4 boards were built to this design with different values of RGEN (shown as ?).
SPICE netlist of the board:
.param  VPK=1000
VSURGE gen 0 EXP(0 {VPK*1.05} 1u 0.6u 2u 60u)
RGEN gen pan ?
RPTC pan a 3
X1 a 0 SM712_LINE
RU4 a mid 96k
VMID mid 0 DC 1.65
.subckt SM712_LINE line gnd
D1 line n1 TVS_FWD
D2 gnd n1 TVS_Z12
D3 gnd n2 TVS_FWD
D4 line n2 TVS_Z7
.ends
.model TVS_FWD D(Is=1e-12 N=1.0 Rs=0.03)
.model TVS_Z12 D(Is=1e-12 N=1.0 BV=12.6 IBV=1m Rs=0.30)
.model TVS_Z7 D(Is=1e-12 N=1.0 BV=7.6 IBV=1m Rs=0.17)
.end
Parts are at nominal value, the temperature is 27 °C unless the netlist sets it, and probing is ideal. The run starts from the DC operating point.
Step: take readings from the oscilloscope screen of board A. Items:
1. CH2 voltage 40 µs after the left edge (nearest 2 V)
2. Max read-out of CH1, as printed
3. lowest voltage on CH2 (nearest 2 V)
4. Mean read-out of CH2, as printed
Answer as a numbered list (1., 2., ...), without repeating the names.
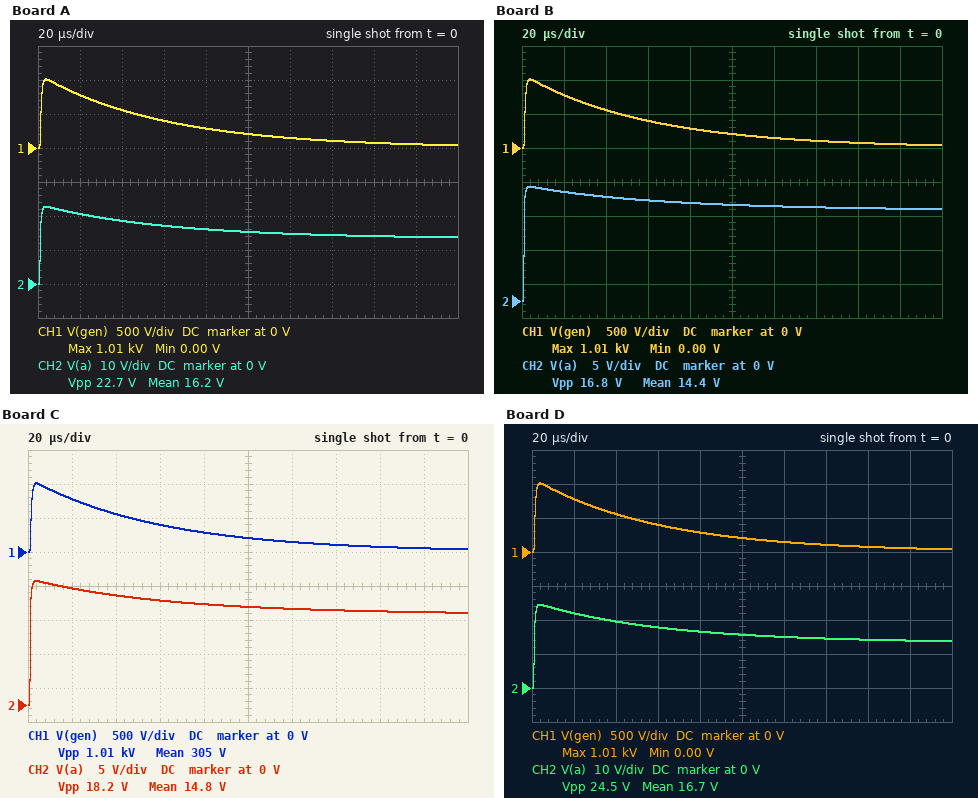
1. 18 V
2. 1.01 kV
3. 0 V
4. 16.2 V
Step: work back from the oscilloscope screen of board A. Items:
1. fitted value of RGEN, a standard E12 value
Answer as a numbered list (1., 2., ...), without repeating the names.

1. 33 Ω
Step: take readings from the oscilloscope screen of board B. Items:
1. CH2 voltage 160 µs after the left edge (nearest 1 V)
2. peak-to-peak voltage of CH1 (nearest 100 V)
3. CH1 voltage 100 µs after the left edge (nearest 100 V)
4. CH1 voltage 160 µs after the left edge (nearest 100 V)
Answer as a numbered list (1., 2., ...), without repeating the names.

1. 14 V
2. 1.0 kV
3. 200 V
4. 100 V
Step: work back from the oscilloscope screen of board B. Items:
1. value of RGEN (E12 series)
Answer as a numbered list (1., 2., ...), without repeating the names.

1. 100 Ω
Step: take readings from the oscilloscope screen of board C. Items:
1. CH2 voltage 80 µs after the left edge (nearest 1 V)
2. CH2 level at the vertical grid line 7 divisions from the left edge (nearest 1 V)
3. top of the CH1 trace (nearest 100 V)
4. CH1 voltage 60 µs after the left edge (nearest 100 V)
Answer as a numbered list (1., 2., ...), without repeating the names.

1. 15 V
2. 14 V
3. 1.0 kV
4. 400 V
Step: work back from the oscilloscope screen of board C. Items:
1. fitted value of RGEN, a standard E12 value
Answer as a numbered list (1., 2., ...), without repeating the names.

1. 68 Ω
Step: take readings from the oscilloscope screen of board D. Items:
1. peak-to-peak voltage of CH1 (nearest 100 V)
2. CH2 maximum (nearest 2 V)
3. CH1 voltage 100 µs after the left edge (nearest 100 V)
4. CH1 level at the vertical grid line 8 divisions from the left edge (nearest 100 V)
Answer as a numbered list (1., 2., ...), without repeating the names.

1. 1.0 kV
2. 24 V
3. 200 V
4. 100 V
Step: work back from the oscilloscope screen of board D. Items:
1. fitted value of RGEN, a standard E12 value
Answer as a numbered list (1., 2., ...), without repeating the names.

1. 27 Ω
